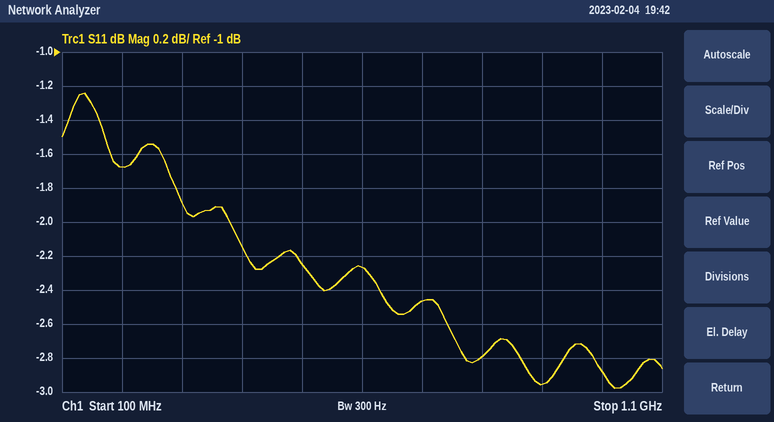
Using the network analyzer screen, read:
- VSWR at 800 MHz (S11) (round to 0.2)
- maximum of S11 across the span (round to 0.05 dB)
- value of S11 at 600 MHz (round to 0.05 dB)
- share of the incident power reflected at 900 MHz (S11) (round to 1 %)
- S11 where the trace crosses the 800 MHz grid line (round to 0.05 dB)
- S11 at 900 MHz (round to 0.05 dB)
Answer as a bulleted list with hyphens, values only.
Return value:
- 6.2
- -1.25 dB
- -2.25 dB
- 51 %
- -2.80 dB
- -2.95 dB
